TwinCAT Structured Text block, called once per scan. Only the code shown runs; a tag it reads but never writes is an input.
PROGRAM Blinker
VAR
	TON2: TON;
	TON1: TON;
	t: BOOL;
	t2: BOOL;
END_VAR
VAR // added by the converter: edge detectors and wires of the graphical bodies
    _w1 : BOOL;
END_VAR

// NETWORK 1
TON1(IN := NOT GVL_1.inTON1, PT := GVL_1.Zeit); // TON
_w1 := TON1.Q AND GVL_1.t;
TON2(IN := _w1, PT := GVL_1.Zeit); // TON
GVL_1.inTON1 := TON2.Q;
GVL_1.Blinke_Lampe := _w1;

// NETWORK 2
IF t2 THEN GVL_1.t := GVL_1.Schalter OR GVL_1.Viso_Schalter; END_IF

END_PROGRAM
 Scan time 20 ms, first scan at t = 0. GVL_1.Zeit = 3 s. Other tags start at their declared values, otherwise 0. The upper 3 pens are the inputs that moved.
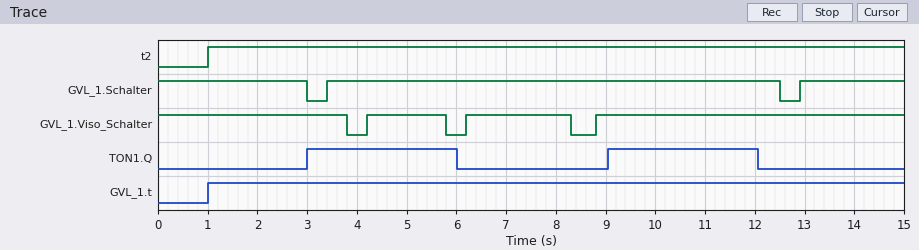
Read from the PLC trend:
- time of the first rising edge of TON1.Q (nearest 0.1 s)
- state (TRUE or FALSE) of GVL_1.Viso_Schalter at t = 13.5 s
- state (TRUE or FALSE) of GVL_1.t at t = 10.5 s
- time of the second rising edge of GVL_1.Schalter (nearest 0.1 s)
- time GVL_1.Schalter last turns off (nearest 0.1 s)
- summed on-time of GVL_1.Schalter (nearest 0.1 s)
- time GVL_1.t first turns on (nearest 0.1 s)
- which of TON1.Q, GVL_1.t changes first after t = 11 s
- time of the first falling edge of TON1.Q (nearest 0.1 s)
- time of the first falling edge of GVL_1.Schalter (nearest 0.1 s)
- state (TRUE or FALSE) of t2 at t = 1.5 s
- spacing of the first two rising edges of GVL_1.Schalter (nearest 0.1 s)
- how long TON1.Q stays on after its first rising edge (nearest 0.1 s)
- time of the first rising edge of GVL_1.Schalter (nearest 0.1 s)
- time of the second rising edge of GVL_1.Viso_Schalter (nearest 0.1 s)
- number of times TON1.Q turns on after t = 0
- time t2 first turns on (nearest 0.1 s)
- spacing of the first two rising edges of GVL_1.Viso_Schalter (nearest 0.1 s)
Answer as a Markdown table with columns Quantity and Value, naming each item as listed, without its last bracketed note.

| Quantity | Value |
|---|---|
| time of the first rising edge of TON1.Q | 3.0 s |
| state (TRUE or FALSE) of GVL_1.Viso_Schalter at t = 13.5 s | TRUE |
| state (TRUE or FALSE) of GVL_1.t at t = 10.5 s | TRUE |
| time of the second rising edge of GVL_1.Schalter | 12.9 s |
| time GVL_1.Schalter last turns off | 12.5 s |
| summed on-time of GVL_1.Schalter | 14.2 s |
| time GVL_1.t first turns on | 1.0 s |
| which of TON1.Q, GVL_1.t changes first after t = 11 s | TON1.Q |
| time of the first falling edge of TON1.Q | 6.0 s |
| time of the first falling edge of GVL_1.Schalter | 3.0 s |
| state (TRUE or FALSE) of t2 at t = 1.5 s | TRUE |
| spacing of the first two rising edges of GVL_1.Schalter | 9.5 s |
| how long TON1.Q stays on after its first rising edge | 3.0 s |
| time of the first rising edge of GVL_1.Schalter | 3.4 s |
| time of the second rising edge of GVL_1.Viso_Schalter | 6.2 s |
| number of times TON1.Q turns on after t = 0 | 2 |
| time t2 first turns on | 1.0 s |
| spacing of the first two rising edges of GVL_1.Viso_Schalter | 2.0 s |
